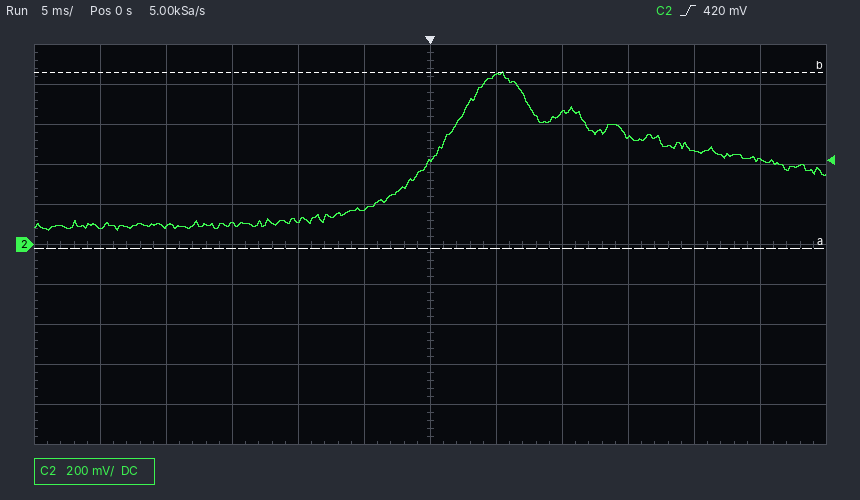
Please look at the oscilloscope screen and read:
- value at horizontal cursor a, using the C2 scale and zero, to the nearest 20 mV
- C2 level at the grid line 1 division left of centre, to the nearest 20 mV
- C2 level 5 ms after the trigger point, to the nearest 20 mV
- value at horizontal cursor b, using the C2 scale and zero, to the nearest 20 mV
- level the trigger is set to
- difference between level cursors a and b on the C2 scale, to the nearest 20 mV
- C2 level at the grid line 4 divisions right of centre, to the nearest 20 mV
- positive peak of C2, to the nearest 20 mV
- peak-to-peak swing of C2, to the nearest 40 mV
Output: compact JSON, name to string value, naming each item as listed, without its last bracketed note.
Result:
{"value at horizontal cursor a, using the C2 scale and zero, to the nearest 20 mV": "-20 mV", "C2 level at the grid line 1 division left of centre, to the nearest 20 mV": "180 mV", "C2 level 5 ms after the trigger point, to the nearest 20 mV": "840 mV", "value at horizontal cursor b, using the C2 scale and zero, to the nearest 20 mV": "860 mV", "level the trigger is set to": "420 mV", "difference between level cursors a and b on the C2 scale, to the nearest 20 mV": "880 mV", "C2 level at the grid line 4 divisions right of centre, to the nearest 20 mV": "460 mV", "positive peak of C2, to the nearest 20 mV": "860 mV", "peak-to-peak swing of C2, to the nearest 40 mV": "800 mV"}
